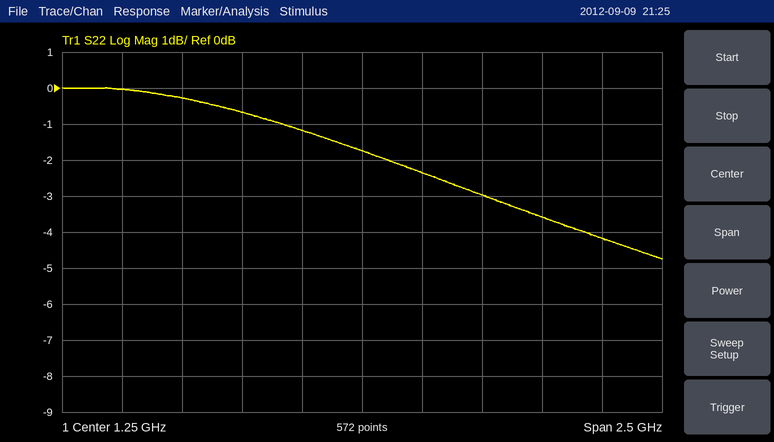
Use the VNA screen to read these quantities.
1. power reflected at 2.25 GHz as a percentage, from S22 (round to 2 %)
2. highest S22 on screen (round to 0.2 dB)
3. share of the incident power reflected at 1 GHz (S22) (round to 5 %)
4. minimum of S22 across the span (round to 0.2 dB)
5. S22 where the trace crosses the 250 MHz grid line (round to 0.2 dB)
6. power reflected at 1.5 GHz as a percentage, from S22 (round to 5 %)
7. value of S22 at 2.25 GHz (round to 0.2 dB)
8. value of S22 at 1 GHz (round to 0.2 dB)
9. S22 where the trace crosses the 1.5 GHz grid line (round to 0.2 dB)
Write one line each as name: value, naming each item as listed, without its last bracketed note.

power reflected at 2.25 GHz as a percentage, from S22: 38 %
highest S22 on screen: 0.0 dB
share of the incident power reflected at 1 GHz (S22): 75 %
minimum of S22 across the span: -4.8 dB
S22 where the trace crosses the 250 MHz grid line: 0.0 dB
power reflected at 1.5 GHz as a percentage, from S22: 60 %
value of S22 at 2.25 GHz: -4.2 dB
value of S22 at 1 GHz: -1.2 dB
S22 where the trace crosses the 1.5 GHz grid line: -2.4 dB
